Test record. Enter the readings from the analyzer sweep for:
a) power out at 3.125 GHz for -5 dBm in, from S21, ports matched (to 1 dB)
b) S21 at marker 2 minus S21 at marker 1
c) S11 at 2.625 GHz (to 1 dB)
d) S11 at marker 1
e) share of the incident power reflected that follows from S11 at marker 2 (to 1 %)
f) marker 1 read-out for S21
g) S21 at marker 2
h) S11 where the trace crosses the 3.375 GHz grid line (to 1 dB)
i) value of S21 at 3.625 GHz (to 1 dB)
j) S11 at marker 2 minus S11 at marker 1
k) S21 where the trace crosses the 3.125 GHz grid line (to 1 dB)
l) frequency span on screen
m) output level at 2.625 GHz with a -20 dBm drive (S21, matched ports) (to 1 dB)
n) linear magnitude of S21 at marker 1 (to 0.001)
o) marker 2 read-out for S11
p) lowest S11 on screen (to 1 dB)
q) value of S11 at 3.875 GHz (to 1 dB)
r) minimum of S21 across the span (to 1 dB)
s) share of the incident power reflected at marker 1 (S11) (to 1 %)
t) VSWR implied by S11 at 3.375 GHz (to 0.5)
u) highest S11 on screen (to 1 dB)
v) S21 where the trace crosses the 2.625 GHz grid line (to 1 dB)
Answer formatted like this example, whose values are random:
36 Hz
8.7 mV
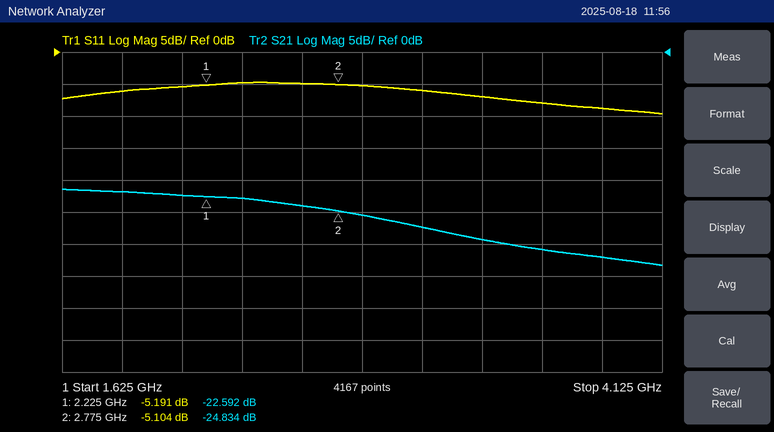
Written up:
-32 dBm
-2.242 dB
-5 dB
-5.191 dB
31 %
-22.592 dB
-24.834 dB
-7 dB
-31 dB
0.087 dB
-27 dB
2.5 GHz
-44 dBm
0.074
-5.104 dB
-10 dB
-9 dB
-33 dB
30 %
2.5
-5 dB
-24 dB
